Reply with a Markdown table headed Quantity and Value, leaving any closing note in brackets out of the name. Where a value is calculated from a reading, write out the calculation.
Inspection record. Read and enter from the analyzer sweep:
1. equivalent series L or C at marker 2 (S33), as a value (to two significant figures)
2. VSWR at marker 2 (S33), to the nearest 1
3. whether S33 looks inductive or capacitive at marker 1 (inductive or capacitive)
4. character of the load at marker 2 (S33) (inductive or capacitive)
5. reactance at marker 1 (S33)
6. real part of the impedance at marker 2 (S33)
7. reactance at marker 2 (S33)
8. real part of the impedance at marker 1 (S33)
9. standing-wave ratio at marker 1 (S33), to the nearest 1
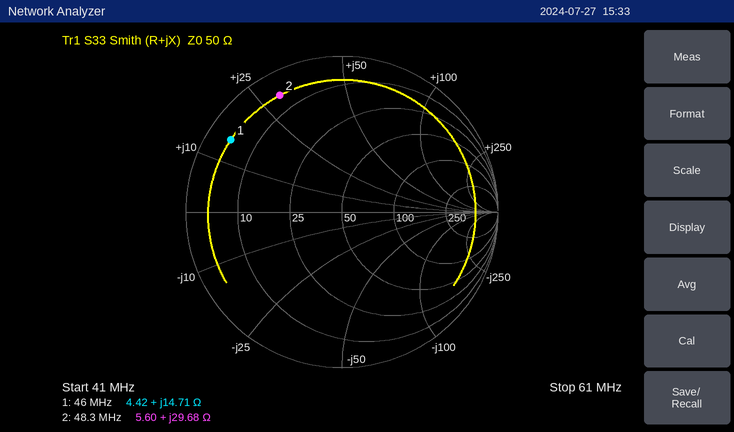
| Quantity | Value |
|---|---|
| equivalent series L or C at marker 2 (S33), as a value | L = 29.68 Ω/(2π × 48.3 MHz) ≈ 98 nH |
| VSWR at marker 2 (S33), to the nearest 1 | 12 |
| whether S33 looks inductive or capacitive at marker 1 | inductive |
| character of the load at marker 2 (S33) | inductive |
| reactance at marker 1 | +14.71 Ω |
| real part of the impedance at marker 2 | 5.60 Ω |
| reactance at marker 2 | +29.68 Ω |
| real part of the impedance at marker 1 | 4.42 Ω |
| standing-wave ratio at marker 1 (S33), to the nearest 1 | 12 |
